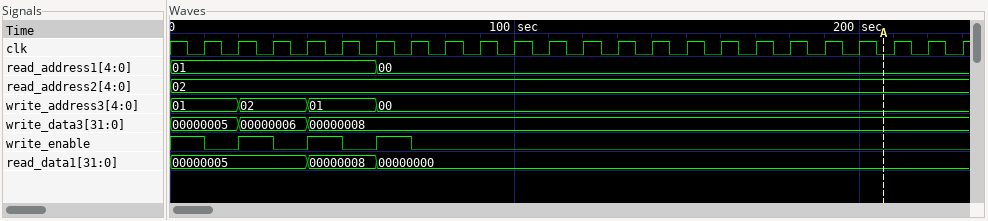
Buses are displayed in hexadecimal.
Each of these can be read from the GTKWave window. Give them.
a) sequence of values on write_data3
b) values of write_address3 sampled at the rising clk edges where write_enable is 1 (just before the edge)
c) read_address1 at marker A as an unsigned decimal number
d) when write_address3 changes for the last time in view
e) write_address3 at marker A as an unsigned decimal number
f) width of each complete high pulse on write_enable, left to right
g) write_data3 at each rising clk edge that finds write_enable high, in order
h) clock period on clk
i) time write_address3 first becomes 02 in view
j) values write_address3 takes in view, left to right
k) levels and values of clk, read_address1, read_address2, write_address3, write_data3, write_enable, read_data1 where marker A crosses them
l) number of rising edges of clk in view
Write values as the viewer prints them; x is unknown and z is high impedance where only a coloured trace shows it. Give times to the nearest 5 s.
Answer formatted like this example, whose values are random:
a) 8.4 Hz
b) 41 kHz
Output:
a) 00000005, 00000006, 00000008
b) 01, 02, 01, 00
c) 0
d) 60 s
e) 0
f) 10 s, 10 s, 10 s
g) 00000005, 00000006, 00000008, 00000008
h) 10 s
i) 20 s
j) 01, 02, 01, 00
k) clk=0, read_address1=00, read_address2=02, write_address3=00, write_data3=00000008, write_enable=0, read_data1=00000000
l) 23
